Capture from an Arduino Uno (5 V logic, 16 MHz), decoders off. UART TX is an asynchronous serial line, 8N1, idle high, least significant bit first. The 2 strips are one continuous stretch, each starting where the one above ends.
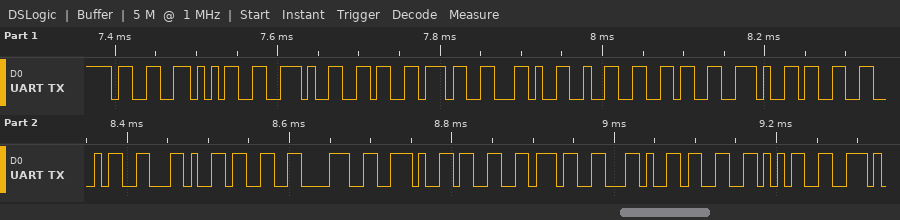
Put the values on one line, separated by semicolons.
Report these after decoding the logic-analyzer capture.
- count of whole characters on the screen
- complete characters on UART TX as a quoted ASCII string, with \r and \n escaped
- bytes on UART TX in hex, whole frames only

20; "35.67,26.34,38.37,35"; 33 35 2E 36 37 2C 32 36 2E 33 34 2C 33 38 2E 33 37 2C 33 35
